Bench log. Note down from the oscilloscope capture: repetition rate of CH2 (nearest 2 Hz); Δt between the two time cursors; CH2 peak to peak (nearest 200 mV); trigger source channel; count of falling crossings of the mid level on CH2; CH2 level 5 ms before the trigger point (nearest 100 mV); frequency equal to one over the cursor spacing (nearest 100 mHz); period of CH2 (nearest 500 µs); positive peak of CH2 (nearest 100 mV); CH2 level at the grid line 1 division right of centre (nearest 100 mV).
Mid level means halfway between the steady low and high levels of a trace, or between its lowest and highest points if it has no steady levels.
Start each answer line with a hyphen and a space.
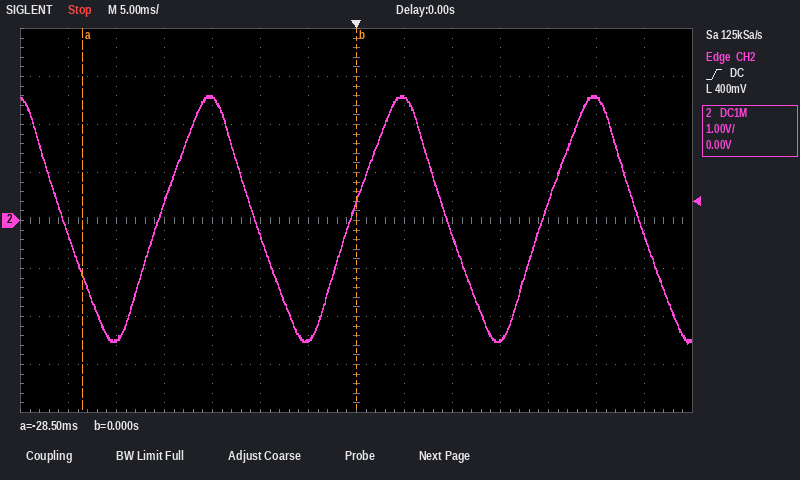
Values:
- 50 Hz
- 28.5 ms
- 5.2 V
- CH2
- 4
- -2.5 V
- 35.1 Hz
- 20.0 ms
- 2.6 V
- 2.6 V
